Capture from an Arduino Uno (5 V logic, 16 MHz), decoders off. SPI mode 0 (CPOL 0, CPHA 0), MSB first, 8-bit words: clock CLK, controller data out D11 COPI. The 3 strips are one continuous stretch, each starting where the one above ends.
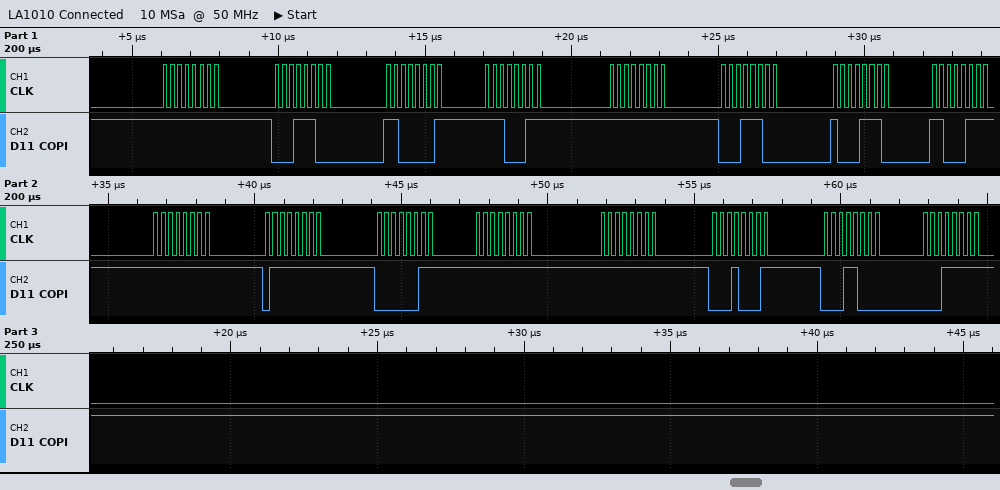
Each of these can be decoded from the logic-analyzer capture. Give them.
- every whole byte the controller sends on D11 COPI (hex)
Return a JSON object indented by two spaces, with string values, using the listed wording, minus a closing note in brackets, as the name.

{
  "every whole byte the controller sends on D11 COPI": "0xFF 0x1C 0xC1 0xE3 0xFF 0x1C 0x8E 0xC7 0xFF 0x7F 0x03 0xFF 0xFF 0x11 0x18 0x1F"
}
